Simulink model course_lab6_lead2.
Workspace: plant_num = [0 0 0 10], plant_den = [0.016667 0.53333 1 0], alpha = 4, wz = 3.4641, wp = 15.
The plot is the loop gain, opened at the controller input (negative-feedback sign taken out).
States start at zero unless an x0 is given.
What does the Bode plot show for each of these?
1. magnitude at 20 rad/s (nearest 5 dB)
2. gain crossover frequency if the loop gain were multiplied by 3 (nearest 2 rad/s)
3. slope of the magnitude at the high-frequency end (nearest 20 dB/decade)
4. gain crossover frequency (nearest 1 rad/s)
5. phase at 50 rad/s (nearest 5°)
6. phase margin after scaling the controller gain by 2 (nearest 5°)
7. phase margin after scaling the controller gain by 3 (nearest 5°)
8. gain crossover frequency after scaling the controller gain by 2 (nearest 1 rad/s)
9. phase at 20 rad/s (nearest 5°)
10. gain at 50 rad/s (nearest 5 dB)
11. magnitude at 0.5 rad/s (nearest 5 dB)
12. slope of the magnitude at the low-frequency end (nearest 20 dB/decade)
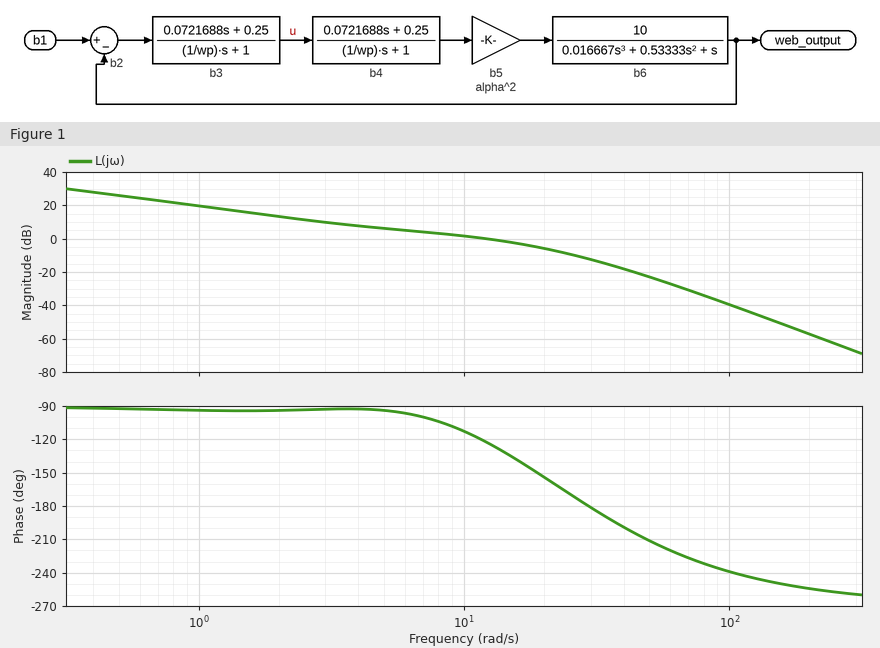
-5 dB
26 rad/s
-60 dB/decade
12 rad/s
-210°
25°
10°
20 rad/s
-155°
-25 dB
25 dB
-20 dB/decade
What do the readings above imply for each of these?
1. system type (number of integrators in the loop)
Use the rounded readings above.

1
